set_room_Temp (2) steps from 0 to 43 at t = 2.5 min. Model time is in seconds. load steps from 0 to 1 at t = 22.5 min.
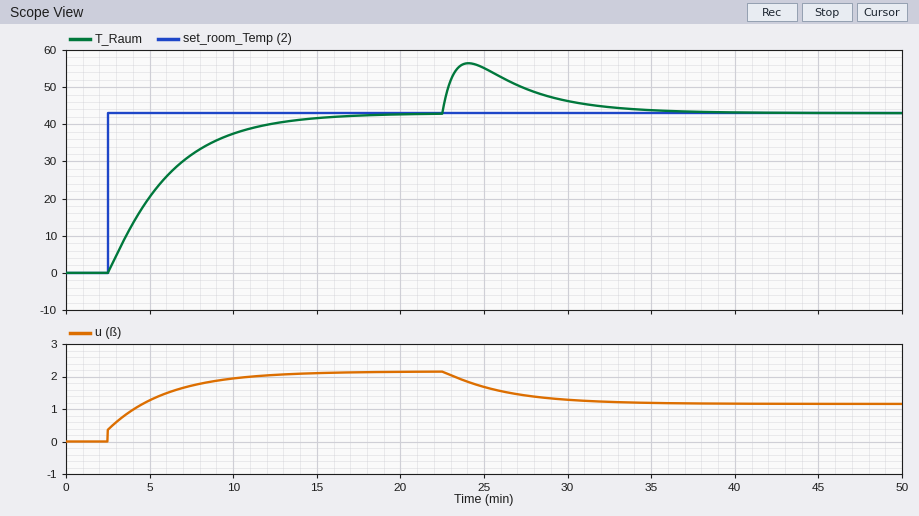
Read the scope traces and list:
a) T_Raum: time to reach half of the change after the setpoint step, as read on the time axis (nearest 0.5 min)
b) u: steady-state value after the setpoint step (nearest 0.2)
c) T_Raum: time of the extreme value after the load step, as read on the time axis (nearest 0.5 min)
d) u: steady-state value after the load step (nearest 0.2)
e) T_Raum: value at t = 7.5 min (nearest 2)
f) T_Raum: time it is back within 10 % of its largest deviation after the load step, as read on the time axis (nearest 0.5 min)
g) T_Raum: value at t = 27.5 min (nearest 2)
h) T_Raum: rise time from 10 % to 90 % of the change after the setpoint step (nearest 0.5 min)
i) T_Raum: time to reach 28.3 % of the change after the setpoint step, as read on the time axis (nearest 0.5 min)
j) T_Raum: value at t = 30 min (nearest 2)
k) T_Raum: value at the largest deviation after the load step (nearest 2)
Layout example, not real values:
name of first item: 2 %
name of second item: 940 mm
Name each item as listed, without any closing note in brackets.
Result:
T_Raum: time to reach half of the change after the setpoint step, as read on the time axis: 5.0 min
u: steady-state value after the setpoint step: 2.2
T_Raum: time of the extreme value after the load step, as read on the time axis: 24.0 min
u: steady-state value after the load step: 1.2
T_Raum: value at t = 7.5 min: 32
T_Raum: time it is back within 10 % of its largest deviation after the load step, as read on the time axis: 33.0 min
T_Raum: value at t = 27.5 min: 50
T_Raum: rise time from 10 % to 90 % of the change after the setpoint step: 8.0 min
T_Raum: time to reach 28.3 % of the change after the setpoint step, as read on the time axis: 4.0 min
T_Raum: value at t = 30 min: 46
T_Raum: value at the largest deviation after the load step: 56
